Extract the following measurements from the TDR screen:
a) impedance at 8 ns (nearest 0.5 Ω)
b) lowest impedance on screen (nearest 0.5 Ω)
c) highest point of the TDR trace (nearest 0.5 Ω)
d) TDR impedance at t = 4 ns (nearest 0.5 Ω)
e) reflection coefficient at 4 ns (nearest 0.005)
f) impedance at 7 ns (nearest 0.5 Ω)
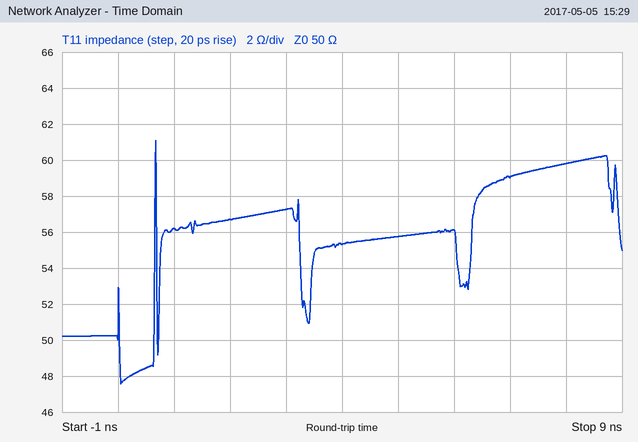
60.0 Ω
47.5 Ω
61.0 Ω
55.5 Ω
+0.050
59.0 Ω
